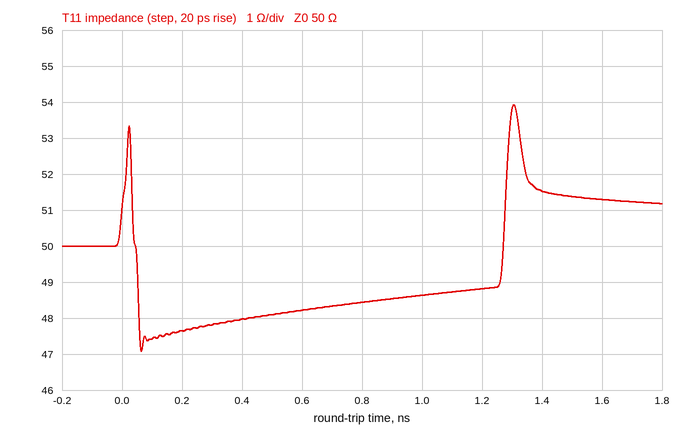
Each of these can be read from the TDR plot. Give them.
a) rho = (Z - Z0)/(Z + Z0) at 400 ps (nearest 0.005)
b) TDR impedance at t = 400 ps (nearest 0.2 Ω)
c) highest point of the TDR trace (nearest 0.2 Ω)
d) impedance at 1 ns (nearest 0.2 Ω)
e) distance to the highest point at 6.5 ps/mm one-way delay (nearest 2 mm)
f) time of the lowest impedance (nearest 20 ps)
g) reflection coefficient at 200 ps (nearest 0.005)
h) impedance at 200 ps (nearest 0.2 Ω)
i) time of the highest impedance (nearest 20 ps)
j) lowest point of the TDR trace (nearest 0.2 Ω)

-0.020
48.0 Ω
54.0 Ω
48.6 Ω
100 mm
60 ps
-0.025
47.6 Ω
1.30 ns
47.0 Ω
